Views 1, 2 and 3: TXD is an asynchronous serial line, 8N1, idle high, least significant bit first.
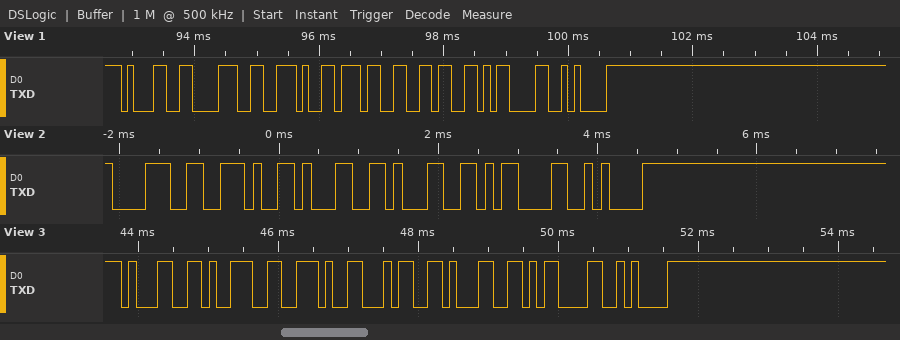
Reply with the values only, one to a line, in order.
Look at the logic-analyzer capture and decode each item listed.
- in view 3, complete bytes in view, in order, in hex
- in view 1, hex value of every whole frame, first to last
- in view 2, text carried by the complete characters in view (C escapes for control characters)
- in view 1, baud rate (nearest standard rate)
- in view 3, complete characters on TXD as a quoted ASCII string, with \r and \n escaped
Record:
31 39 2E 34 31 0D 0A
0x31 0x38 0x2E 0x37 0x36 0x0D 0x0A
"8.11\r\n"
9600 baud
"19.41\r\n"
